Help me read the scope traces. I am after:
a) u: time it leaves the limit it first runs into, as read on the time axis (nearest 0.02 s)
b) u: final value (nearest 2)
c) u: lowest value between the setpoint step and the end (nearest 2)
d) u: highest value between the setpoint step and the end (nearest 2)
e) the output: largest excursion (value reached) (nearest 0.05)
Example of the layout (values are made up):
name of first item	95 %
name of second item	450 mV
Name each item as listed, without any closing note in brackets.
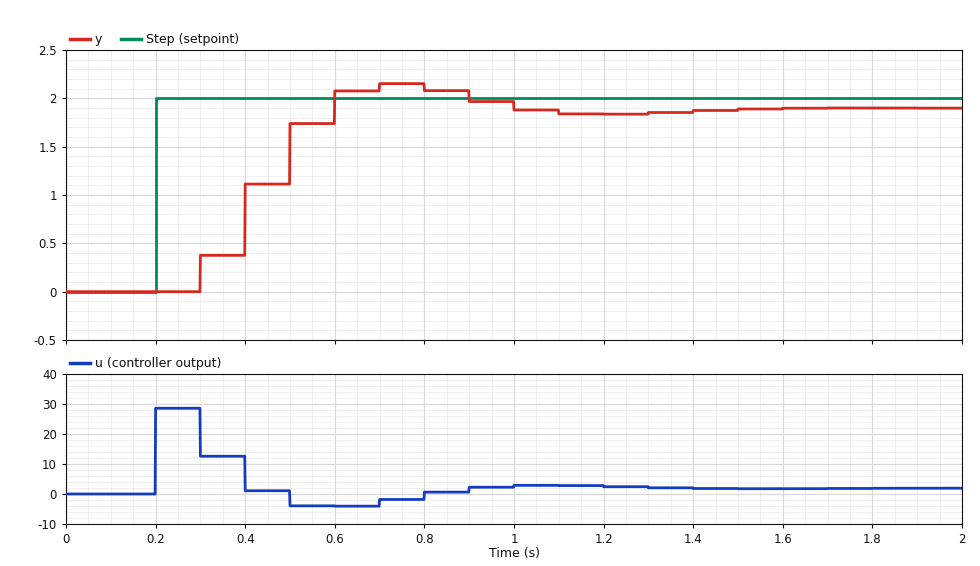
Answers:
u: time it leaves the limit it first runs into, as read on the time axis	0.30 s
u: final value	2
u: lowest value between the setpoint step and the end	-4
u: highest value between the setpoint step and the end	28
the output: largest excursion (value reached)	2.15
